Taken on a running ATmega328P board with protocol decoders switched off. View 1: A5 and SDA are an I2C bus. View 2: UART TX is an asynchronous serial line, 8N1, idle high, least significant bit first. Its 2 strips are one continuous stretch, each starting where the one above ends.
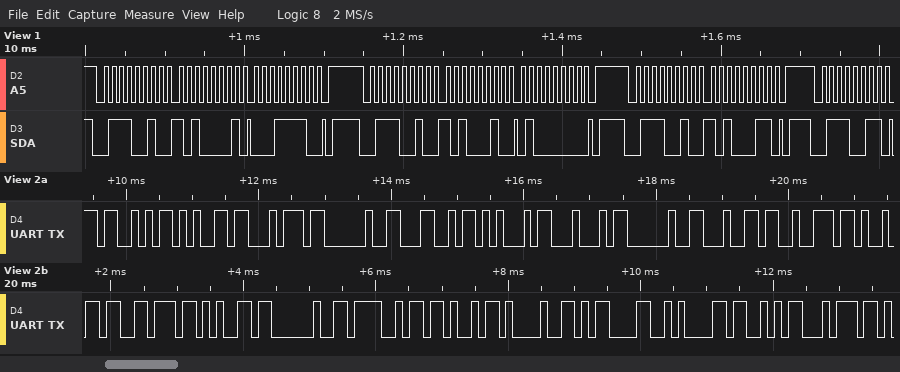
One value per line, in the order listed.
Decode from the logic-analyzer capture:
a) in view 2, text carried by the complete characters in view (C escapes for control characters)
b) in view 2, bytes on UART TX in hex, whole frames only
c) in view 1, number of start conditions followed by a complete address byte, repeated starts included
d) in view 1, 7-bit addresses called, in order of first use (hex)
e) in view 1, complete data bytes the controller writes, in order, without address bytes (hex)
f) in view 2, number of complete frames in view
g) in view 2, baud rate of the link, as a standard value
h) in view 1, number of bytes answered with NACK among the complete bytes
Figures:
"Set LED drive OK!\r\nSt"
0x53 0x65 0x74 0x20 0x4C 0x45 0x44 0x20 0x64 0x72 0x69 0x76 0x65 0x20 0x4F 0x4B 0x21 0x0D 0x0A 0x53 0x74
4
0x39
A1 1E A2 40 A3
21
9600 baud
0
